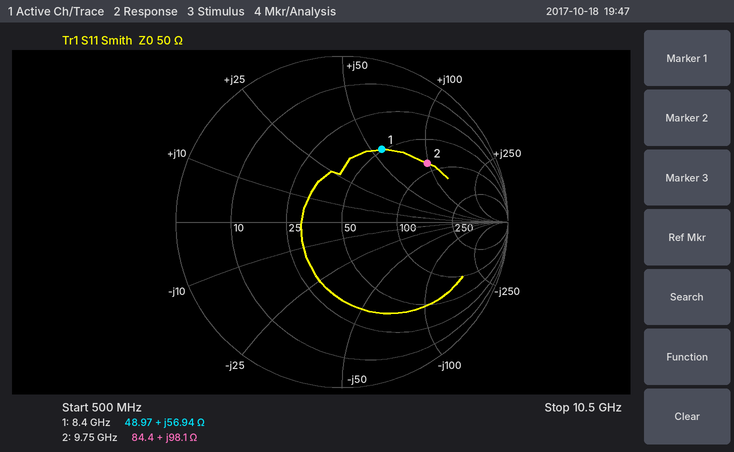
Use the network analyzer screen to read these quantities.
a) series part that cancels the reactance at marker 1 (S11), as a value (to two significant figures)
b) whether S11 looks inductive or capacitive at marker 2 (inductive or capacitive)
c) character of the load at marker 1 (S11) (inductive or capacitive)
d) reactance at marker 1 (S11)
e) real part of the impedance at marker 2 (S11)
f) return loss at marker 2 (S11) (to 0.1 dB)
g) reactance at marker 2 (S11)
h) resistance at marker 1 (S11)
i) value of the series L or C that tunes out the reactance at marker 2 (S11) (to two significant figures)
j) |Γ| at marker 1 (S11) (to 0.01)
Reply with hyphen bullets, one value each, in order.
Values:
- 330 fF
- inductive
- inductive
- +56.94 Ω
- 84.4 Ω
- 4.1 dB
- +98.1 Ω
- 48.97 Ω
- 170 fF
- 0.50
